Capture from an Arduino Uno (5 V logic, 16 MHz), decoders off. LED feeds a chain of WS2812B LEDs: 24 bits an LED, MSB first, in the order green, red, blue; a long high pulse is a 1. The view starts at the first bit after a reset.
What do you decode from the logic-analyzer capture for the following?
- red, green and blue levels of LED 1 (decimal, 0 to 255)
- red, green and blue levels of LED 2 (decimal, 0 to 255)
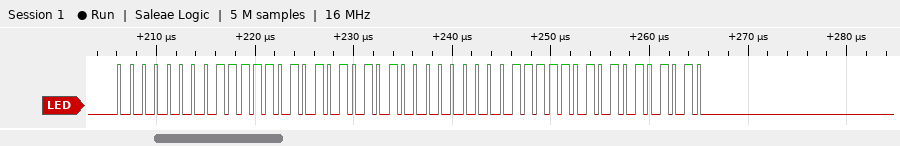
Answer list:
250, 0, 170
250, 0, 170
